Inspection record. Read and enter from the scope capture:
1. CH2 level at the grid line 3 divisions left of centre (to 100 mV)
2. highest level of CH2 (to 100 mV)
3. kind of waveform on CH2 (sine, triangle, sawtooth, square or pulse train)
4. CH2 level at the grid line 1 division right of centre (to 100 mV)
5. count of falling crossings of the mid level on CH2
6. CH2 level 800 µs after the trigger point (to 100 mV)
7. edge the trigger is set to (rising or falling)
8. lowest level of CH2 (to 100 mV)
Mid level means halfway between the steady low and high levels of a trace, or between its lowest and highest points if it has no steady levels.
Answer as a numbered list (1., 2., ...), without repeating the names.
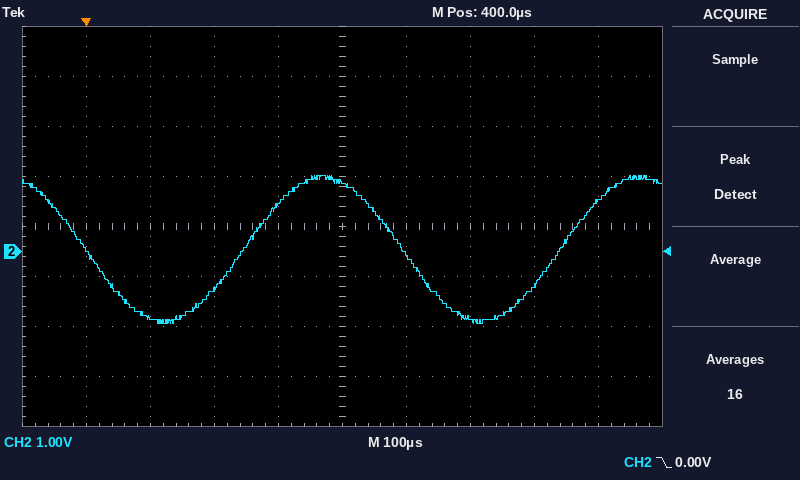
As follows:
1. -1.3 V
2. 1.5 V
3. sine
4. -100 mV
5. 2
6. 1.0 V
7. falling
8. -1.4 V
